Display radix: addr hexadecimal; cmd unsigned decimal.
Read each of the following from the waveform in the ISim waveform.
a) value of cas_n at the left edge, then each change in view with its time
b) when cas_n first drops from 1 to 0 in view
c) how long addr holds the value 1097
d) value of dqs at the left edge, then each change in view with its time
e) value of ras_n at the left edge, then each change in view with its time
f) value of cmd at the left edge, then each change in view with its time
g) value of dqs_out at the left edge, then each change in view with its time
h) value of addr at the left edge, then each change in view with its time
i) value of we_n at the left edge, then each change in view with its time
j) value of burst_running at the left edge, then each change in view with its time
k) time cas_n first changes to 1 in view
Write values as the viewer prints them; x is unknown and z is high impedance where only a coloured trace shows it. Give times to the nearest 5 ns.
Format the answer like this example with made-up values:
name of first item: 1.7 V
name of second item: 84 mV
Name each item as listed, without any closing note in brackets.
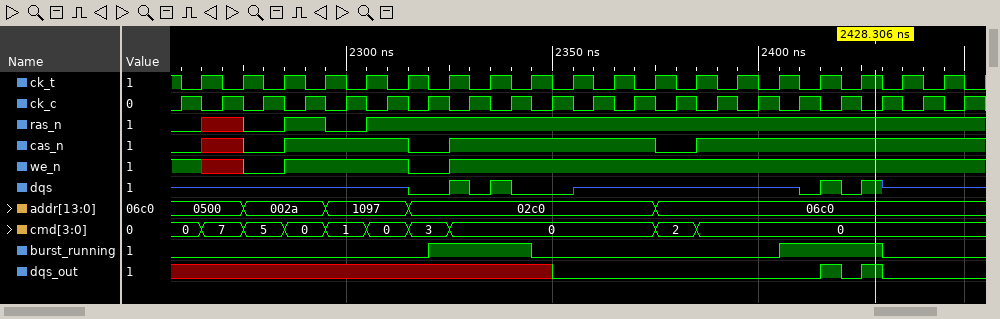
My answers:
value of cas_n at the left edge, then each change in view with its time: 0, x at 2265 ns, 0 at 2275 ns, 1 at 2285 ns, 0 at 2315 ns, 1 at 2325 ns, 0 at 2375 ns, 1 at 2385 ns
when cas_n first drops from 1 to 0 in view: 2315 ns
how long addr holds the value 1097: 20 ns
value of dqs at the left edge, then each change in view with its time: z, 0 at 2315 ns, 1 at 2325 ns, 0 at 2330 ns, 1 at 2335 ns, 0 at 2340 ns, z at 2355 ns, 0 at 2410 ns, 1 at 2415 ns, 0 at 2420 ns, 1 at 2425 ns, z at 2430 ns
value of ras_n at the left edge, then each change in view with its time: 0, x at 2265 ns, 0 at 2275 ns, 1 at 2285 ns, 0 at 2295 ns, 1 at 2305 ns
value of cmd at the left edge, then each change in view with its time: 0, 7 at 2265 ns, 5 at 2275 ns, 0 at 2285 ns, 1 at 2295 ns, 0 at 2305 ns, 3 at 2315 ns, 0 at 2325 ns, 2 at 2375 ns, 0 at 2385 ns
value of dqs_out at the left edge, then each change in view with its time: x, 0 at 2350 ns, 1 at 2415 ns, 0 at 2420 ns, 1 at 2425 ns, 0 at 2430 ns
value of addr at the left edge, then each change in view with its time: 0500, 002a at 2275 ns, 1097 at 2295 ns, 02c0 at 2315 ns, 06c0 at 2375 ns
value of we_n at the left edge, then each change in view with its time: 1, x at 2265 ns, 0 at 2275 ns, 1 at 2285 ns, 0 at 2315 ns, 1 at 2325 ns
value of burst_running at the left edge, then each change in view with its time: 0, 1 at 2320 ns, 0 at 2345 ns, 1 at 2405 ns, 0 at 2430 ns
time cas_n first changes to 1 in view: 2285 ns
